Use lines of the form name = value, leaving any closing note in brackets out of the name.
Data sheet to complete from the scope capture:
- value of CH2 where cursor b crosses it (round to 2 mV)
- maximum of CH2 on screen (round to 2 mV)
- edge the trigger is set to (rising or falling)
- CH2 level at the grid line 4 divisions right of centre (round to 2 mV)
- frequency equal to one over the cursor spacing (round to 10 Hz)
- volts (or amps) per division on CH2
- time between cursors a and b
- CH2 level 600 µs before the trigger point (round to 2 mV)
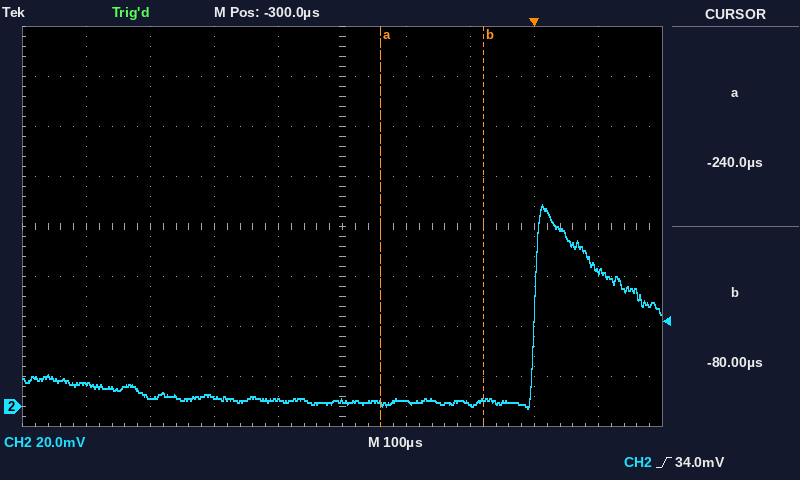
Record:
value of CH2 where cursor b crosses it = 2 mV
maximum of CH2 on screen = 80 mV
edge the trigger is set to = rising
CH2 level at the grid line 4 divisions right of centre = 54 mV
frequency equal to one over the cursor spacing = 6.25 kHz
volts (or amps) per division on CH2 = 20 mV
time between cursors a and b = 160 µs
CH2 level 600 µs before the trigger point = 4 mV
